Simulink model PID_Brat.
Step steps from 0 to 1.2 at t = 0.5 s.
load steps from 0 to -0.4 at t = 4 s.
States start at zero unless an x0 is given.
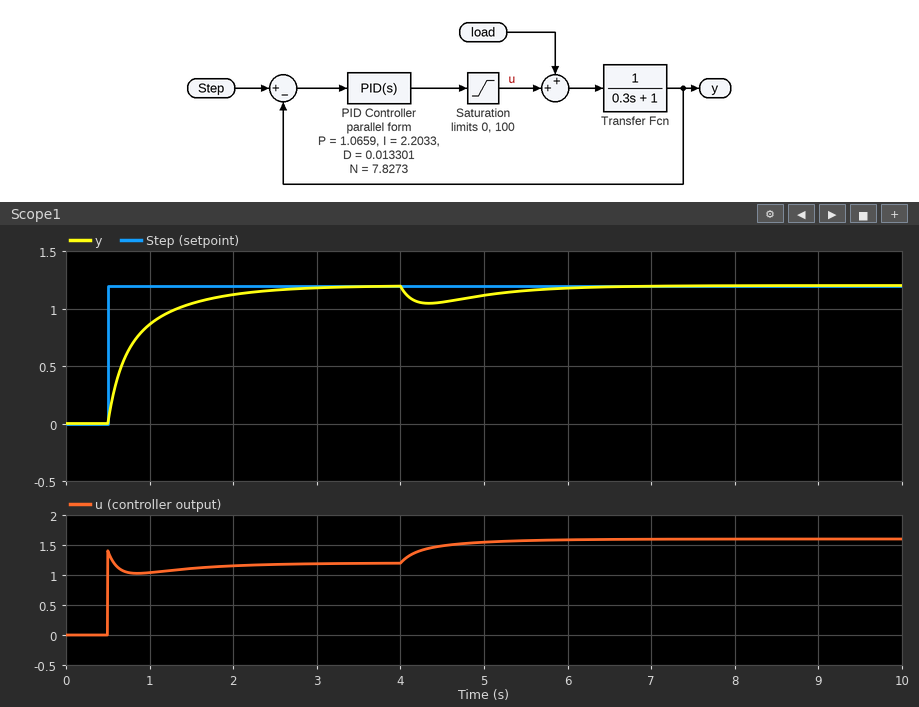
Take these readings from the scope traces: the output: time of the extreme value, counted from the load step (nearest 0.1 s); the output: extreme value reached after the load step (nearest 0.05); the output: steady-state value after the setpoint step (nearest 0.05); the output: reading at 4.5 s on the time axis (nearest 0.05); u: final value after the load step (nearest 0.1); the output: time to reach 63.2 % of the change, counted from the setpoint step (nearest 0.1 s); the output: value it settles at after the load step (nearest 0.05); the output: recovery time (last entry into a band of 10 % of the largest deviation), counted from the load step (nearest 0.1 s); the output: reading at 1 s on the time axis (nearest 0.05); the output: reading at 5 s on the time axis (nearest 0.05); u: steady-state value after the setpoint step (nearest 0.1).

0.3 s
1.05
1.20
1.05
1.6
0.4 s
1.20
2.3 s
0.85
1.10
1.2
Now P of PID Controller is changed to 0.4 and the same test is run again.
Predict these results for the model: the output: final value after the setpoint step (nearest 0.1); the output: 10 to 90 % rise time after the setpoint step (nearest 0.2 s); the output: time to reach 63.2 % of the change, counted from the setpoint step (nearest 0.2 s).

1.2
1.0 s
0.6 s
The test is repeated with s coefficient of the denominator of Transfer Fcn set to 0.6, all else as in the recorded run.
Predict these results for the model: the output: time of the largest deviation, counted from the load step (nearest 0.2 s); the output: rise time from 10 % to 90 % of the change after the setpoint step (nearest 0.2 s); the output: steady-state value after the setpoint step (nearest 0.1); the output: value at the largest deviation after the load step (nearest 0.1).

0.6 s
1.0 s
1.2
1.1
